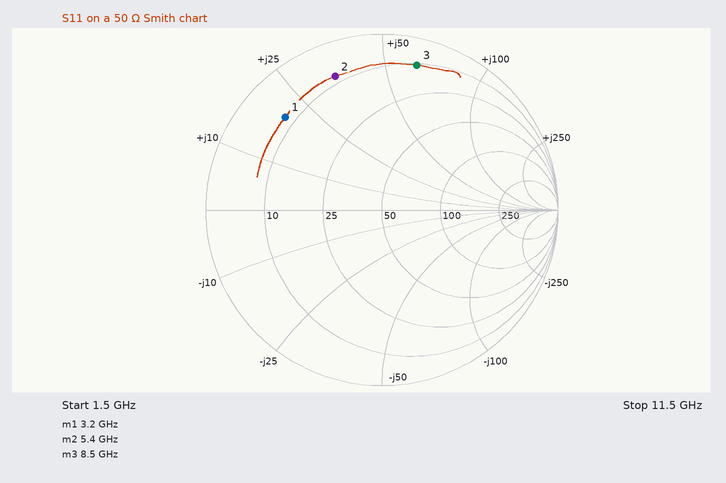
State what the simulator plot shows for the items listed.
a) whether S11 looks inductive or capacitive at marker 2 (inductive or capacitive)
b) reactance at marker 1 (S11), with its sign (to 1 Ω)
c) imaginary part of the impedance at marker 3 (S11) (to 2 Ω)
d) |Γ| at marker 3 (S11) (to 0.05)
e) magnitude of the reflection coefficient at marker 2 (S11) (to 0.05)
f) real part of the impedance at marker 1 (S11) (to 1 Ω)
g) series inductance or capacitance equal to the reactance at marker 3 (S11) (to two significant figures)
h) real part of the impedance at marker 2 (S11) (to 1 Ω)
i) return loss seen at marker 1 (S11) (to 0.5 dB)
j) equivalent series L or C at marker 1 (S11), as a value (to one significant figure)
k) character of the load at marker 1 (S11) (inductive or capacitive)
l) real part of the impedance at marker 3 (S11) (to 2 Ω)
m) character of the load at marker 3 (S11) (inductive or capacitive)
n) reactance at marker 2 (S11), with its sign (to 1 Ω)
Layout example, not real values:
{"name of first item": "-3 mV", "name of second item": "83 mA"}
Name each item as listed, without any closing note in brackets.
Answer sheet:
{"whether S11 looks inductive or capacitive at marker 2": "inductive", "reactance at marker 1 (S11), with its sign": "+20 Ω", "imaginary part of the impedance at marker 3 (S11)": "+62 Ω", "|Γ| at marker 3 (S11)": "0.85", "magnitude of the reflection coefficient at marker 2 (S11)": "0.80", "real part of the impedance at marker 1 (S11)": "8 Ω", "series inductance or capacitance equal to the reactance at marker 3 (S11)": "1.2 nH", "real part of the impedance at marker 2 (S11)": "8 Ω", "return loss seen at marker 1 (S11)": "2.5 dB", "equivalent series L or C at marker 1 (S11), as a value": "1.0 nH", "character of the load at marker 1 (S11)": "inductive", "real part of the impedance at marker 3 (S11)": "10 Ω", "character of the load at marker 3 (S11)": "inductive", "reactance at marker 2 (S11), with its sign": "+35 Ω"}
